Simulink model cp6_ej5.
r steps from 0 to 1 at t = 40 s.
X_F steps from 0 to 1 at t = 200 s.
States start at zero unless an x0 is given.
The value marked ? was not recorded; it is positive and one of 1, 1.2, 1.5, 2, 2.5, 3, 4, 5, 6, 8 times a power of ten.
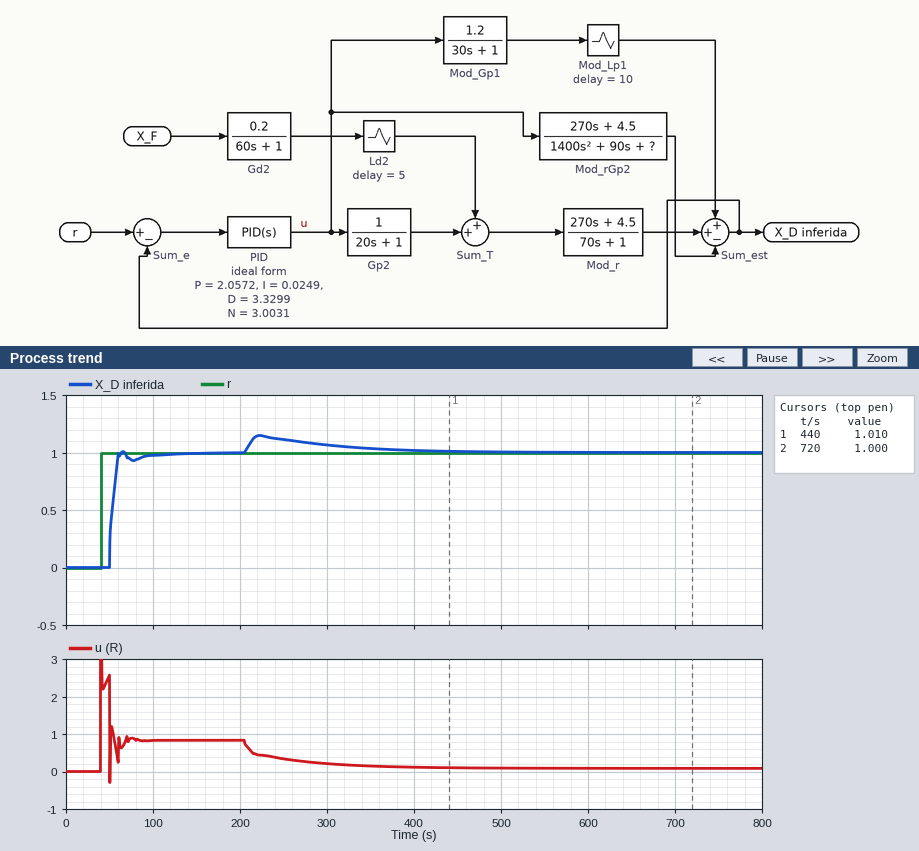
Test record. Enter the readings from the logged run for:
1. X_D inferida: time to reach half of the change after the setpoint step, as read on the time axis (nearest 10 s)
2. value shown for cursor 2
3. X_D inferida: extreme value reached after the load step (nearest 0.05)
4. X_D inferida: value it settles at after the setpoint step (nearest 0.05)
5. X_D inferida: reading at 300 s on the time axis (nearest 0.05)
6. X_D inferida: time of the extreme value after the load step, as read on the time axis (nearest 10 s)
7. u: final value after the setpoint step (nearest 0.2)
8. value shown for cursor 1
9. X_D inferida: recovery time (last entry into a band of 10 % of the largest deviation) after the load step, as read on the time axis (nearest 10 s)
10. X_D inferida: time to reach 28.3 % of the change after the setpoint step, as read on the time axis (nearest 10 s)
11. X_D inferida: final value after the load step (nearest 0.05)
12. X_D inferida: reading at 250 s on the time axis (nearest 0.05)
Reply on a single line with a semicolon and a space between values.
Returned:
50 s; 1.000; 1.15; 1.00; 1.05; 220 s; 0.8; 1.010; 410 s; 50 s; 1.00; 1.10
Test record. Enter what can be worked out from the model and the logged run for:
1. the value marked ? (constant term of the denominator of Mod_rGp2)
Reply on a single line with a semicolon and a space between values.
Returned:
1
